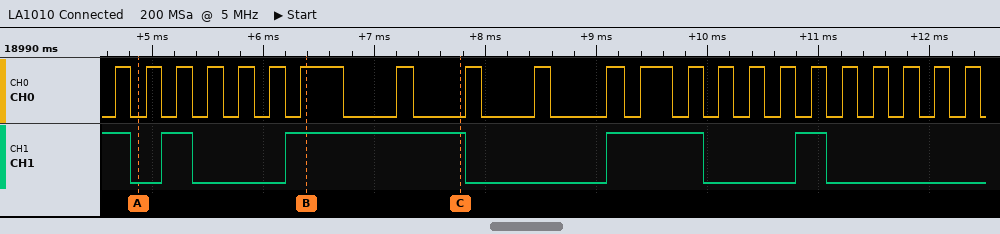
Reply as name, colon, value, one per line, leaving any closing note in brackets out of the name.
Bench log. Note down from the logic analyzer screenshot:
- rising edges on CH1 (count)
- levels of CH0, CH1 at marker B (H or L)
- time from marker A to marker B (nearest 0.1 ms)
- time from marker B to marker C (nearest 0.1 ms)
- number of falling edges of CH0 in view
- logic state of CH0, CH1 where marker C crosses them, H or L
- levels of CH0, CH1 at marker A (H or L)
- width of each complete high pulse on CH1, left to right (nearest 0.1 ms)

rising edges on CH1: 4
levels of CH0, CH1 at marker B: CH0=H, CH1=H
time from marker A to marker B: 1.5 ms
time from marker B to marker C: 1.4 ms
number of falling edges of CH0 in view: 22
logic state of CH0, CH1 where marker C crosses them, H or L: CH0=L, CH1=H
levels of CH0, CH1 at marker A: CH0=L, CH1=L
width of each complete high pulse on CH1, left to right: 0.3 ms, 1.6 ms, 0.9 ms, 0.3 ms
